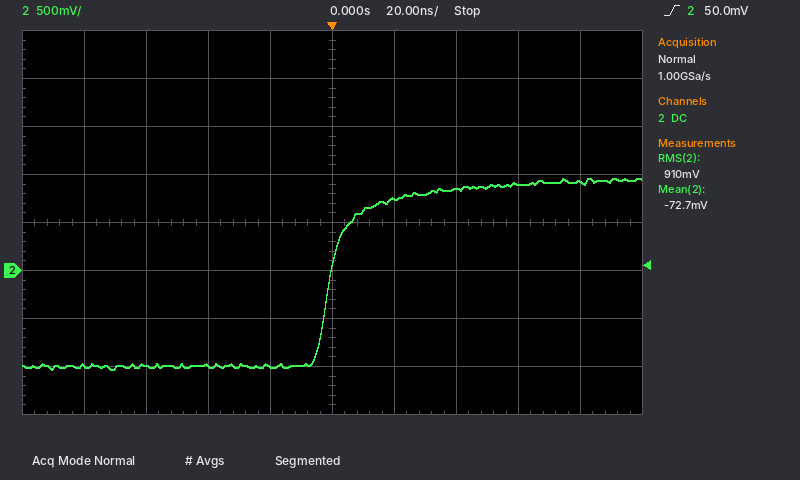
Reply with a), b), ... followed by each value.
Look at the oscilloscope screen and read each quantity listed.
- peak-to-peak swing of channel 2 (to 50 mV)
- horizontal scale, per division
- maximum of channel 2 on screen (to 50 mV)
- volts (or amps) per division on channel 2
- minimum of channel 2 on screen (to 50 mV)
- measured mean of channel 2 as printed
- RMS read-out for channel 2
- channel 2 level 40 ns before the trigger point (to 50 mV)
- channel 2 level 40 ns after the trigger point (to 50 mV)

a) 2.00 V
b) 20 ns
c) 950 mV
d) 500 mV
e) -1.05 V
f) -72.7 mV
g) 910 mV
h) -1.00 V
i) 850 mV
